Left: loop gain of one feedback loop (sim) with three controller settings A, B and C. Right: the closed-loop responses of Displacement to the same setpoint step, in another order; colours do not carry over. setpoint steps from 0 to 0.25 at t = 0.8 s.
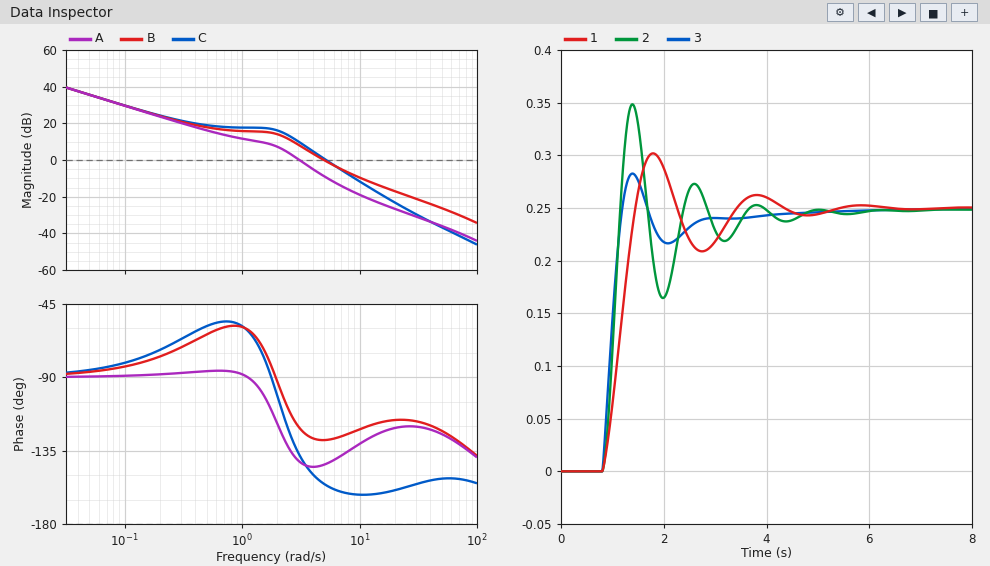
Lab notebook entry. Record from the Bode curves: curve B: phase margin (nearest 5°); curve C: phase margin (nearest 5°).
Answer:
50°
25°
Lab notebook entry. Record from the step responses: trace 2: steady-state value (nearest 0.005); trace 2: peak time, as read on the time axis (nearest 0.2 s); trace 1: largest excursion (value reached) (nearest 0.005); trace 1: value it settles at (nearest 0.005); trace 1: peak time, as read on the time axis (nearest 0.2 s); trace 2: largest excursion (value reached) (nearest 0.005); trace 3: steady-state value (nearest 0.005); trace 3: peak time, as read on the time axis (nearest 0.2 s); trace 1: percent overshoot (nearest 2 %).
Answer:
0.250
1.4 s
0.300
0.250
1.8 s
0.350
0.250
1.4 s
20 %
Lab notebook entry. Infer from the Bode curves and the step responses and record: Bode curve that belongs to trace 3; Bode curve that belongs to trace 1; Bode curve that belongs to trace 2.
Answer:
B
A
C
